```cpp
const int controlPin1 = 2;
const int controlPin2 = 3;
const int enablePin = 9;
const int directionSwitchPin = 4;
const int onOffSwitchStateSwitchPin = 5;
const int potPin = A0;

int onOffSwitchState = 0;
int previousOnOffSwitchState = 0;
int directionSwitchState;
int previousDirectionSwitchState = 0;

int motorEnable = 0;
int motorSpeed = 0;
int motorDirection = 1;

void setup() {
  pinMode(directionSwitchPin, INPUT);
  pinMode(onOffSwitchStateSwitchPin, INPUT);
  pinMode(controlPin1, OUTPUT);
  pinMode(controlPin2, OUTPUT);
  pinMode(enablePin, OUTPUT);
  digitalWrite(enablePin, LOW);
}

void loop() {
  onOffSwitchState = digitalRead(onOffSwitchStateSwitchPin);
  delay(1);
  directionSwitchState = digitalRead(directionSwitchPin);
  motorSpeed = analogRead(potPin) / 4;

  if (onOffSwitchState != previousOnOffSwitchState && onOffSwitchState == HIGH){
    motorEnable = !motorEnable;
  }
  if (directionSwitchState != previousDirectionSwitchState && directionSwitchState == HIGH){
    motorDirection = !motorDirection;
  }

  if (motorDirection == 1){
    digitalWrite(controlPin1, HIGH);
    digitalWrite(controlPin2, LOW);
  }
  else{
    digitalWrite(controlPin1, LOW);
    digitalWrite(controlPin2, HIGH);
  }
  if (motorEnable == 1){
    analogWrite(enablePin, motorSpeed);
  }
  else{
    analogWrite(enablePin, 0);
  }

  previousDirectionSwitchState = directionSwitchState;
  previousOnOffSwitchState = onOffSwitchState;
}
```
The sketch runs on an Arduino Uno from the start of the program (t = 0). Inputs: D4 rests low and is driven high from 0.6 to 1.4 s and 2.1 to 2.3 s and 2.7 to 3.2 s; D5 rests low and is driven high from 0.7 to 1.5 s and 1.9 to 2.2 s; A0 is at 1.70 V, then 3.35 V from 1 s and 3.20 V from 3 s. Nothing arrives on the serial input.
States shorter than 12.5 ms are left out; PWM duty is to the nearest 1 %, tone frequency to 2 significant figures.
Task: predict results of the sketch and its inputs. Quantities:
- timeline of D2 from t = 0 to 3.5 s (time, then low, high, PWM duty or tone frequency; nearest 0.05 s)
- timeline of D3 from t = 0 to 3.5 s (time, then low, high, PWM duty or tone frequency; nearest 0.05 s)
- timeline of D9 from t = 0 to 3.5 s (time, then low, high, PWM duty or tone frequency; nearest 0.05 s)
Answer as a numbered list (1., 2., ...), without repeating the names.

1. 0 s high; 0.6 s low; 2.1 s high; 2.7 s low
2. 0 s low; 0.6 s high; 2.1 s low; 2.7 s high
3. 0 s low; 0.7 s PWM 34 %; 1 s PWM 67 %; 1.9 s low
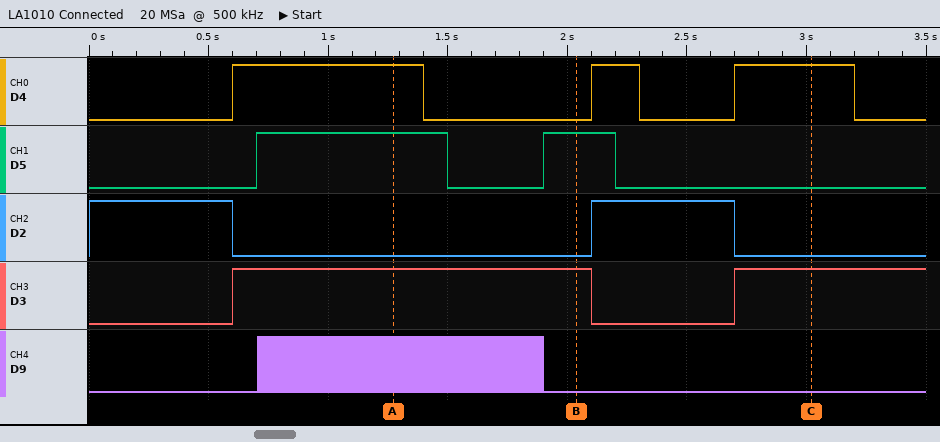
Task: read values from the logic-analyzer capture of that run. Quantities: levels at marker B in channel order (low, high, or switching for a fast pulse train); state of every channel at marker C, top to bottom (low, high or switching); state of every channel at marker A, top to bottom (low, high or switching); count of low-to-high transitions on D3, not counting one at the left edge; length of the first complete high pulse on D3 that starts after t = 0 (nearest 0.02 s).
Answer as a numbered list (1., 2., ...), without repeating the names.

1. D4 low, D5 high, D2 low, D3 high, D9 low
2. D4 high, D5 low, D2 low, D3 high, D9 low
3. D4 high, D5 high, D2 low, D3 high, D9 switching
4. 2
5. 1.50 s
